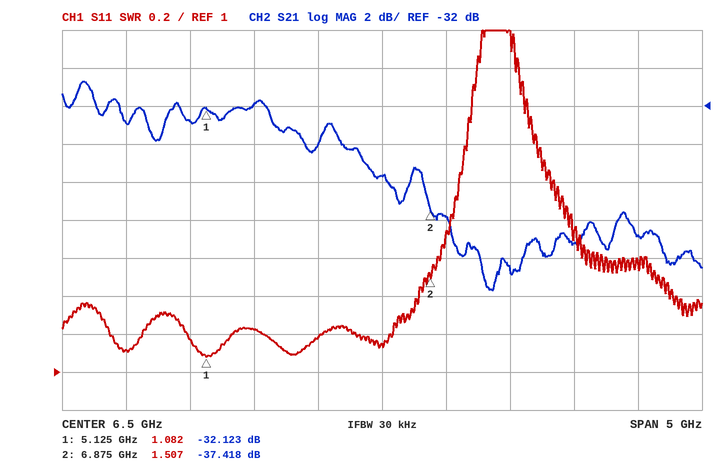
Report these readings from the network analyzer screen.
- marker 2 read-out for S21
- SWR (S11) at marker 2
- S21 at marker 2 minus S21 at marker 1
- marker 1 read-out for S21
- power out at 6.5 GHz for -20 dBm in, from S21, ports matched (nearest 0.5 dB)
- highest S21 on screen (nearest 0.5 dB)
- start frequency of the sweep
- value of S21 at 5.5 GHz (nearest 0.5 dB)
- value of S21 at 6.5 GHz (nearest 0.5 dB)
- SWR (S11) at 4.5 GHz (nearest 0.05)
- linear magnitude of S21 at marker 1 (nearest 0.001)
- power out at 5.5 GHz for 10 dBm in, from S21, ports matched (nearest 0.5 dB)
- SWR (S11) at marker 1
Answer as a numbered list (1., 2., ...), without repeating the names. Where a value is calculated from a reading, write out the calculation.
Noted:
1. -37.418 dB
2. 1.507
3. -37.418 − (-32.123) = -5.295 dB
4. -32.123 dB
5. -20 dBm + (-35.5 dB) = -55.5 dBm
6. -30.5 dB
7. 4 GHz
8. -32.0 dB
9. -35.5 dB
10. 1.10
11. 10^(-32.123/20) ≈ 0.025
12. 10 dBm + (-32.0 dB) = -22.0 dBm
13. 1.082
